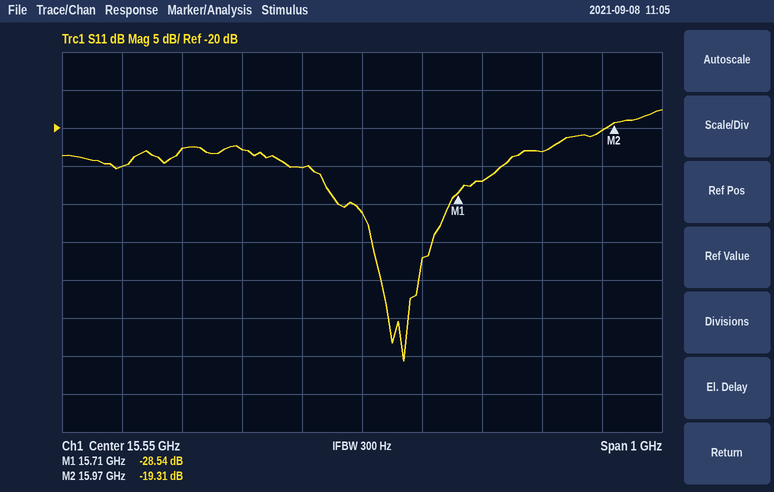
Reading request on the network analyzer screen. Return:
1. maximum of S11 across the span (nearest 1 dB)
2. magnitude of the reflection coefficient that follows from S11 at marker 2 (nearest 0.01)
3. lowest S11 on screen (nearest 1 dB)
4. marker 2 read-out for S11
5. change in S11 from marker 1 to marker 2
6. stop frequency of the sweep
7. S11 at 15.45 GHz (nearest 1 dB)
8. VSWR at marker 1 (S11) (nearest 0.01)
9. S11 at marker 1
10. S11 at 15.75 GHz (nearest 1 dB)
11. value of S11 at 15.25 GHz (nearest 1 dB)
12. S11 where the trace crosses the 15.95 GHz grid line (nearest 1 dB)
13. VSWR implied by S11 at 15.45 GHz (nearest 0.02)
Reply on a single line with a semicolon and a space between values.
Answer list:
-18 dB; 0.11; -51 dB; -19.31 dB; 9.23 dB; 16.05 GHz; -25 dB; 1.08; -28.54 dB; -27 dB; -23 dB; -20 dB; 1.12
